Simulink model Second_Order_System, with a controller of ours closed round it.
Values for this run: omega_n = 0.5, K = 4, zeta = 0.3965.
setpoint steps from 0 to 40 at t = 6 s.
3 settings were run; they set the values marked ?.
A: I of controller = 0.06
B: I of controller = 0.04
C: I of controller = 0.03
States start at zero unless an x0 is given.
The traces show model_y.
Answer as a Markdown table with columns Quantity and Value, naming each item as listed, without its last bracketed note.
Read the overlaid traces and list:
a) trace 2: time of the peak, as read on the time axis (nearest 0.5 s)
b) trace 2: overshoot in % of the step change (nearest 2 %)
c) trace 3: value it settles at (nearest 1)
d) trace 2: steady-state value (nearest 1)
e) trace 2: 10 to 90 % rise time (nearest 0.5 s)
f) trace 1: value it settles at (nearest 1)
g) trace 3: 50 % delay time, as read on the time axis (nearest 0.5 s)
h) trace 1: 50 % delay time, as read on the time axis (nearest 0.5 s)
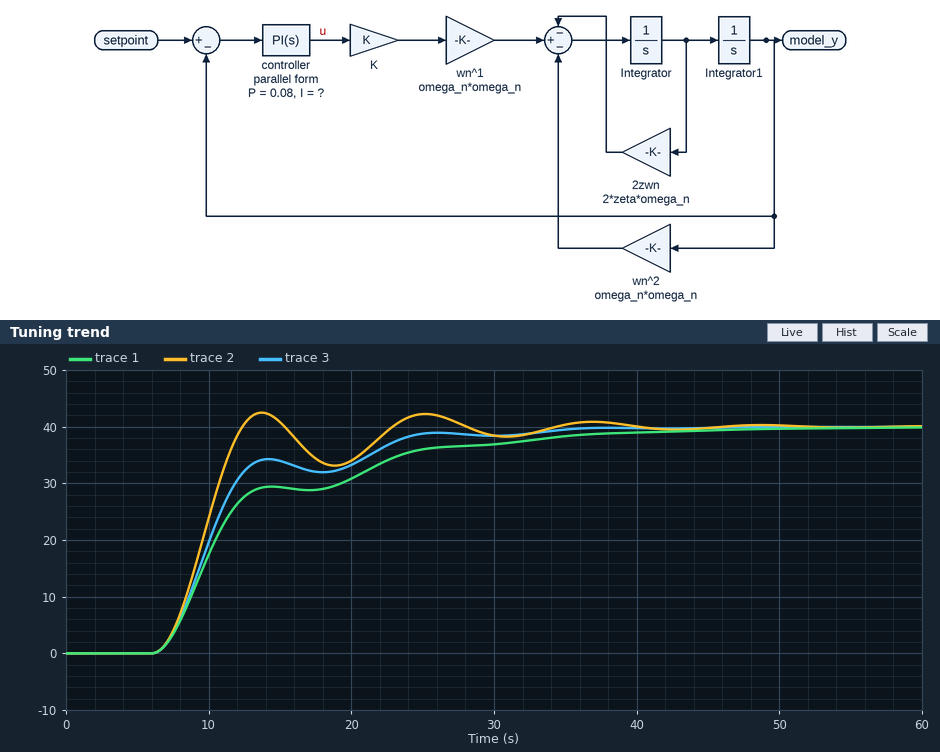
| Quantity | Value |
|---|---|
| trace 2: time of the peak, as read on the time axis | 13.5 s |
| trace 2: overshoot in % of the step change | 6 % |
| trace 3: value it settles at | 40 |
| trace 2: steady-state value | 40 |
| trace 2: 10 to 90 % rise time | 4.0 s |
| trace 1: value it settles at | 40 |
| trace 3: 50 % delay time, as read on the time axis | 10.0 s |
| trace 1: 50 % delay time, as read on the time axis | 10.5 s |
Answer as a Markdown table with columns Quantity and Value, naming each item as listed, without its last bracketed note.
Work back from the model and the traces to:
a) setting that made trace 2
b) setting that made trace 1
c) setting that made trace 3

| Quantity | Value |
|---|---|
| setting that made trace 2 | A |
| setting that made trace 1 | C |
| setting that made trace 3 | B |
